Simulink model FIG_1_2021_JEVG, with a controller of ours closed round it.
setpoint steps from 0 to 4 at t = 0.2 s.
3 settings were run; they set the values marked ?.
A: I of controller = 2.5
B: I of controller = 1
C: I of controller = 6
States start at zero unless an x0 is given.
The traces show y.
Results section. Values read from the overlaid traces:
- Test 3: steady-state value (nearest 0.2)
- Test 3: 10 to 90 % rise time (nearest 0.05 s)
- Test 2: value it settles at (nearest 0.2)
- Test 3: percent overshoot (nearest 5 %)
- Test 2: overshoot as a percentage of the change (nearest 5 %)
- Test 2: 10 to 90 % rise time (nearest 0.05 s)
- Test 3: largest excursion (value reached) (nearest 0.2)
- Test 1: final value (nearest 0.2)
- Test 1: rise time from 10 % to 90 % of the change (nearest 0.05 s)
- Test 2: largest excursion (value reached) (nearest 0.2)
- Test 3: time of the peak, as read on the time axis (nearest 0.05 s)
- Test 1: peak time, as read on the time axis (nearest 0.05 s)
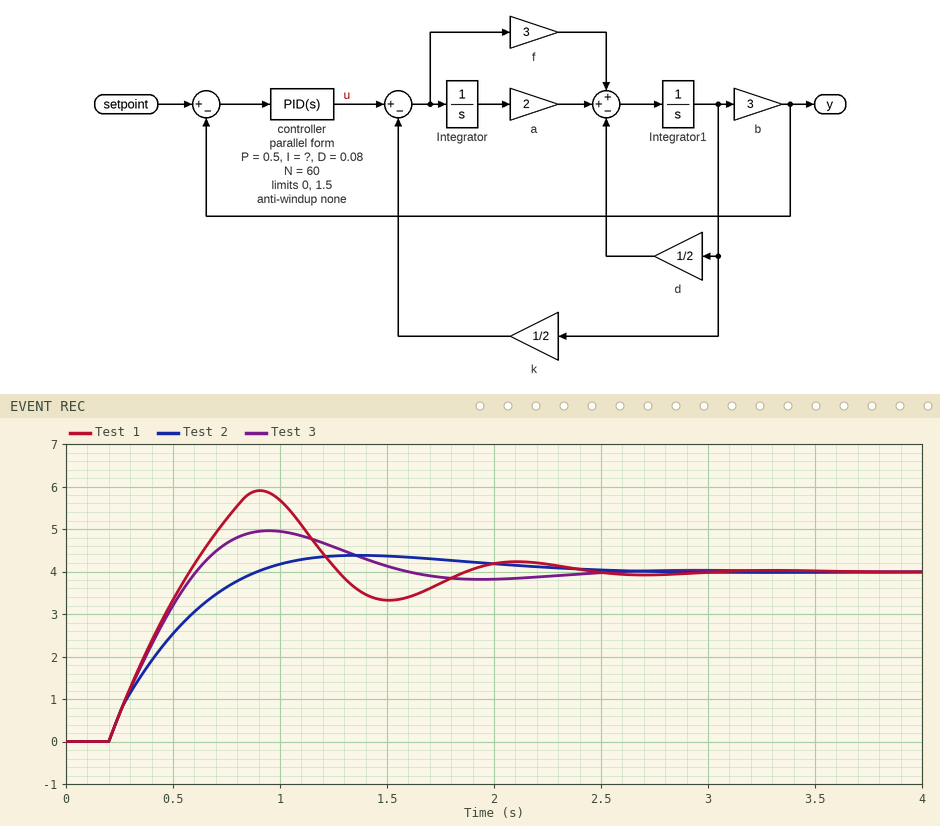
4.0
0.30 s
4.0
25 %
10 %
0.50 s
5.0
4.0
0.30 s
4.4
0.95 s
0.90 s
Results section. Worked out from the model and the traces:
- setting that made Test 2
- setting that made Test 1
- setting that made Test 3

B
C
A
